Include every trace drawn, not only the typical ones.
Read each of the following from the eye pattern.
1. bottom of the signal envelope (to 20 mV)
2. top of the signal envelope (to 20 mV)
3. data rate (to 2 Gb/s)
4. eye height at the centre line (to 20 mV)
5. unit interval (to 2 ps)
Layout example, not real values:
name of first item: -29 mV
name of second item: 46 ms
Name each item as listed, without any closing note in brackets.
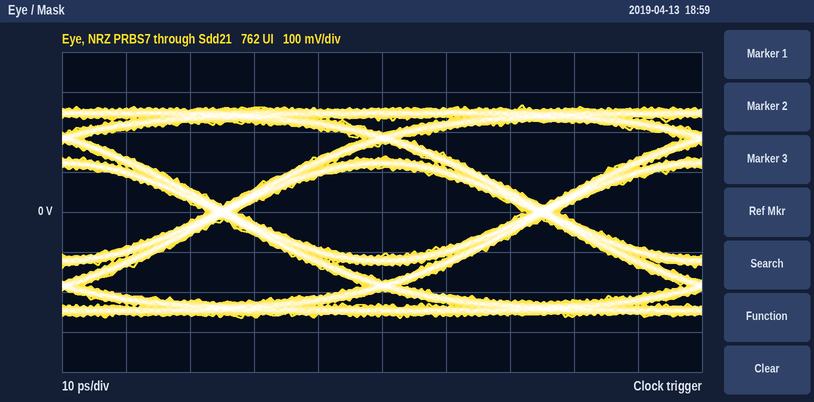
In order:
bottom of the signal envelope: -260 mV
top of the signal envelope: 260 mV
data rate: 20 Gb/s
eye height at the centre line: 220 mV
unit interval: 50 ps
